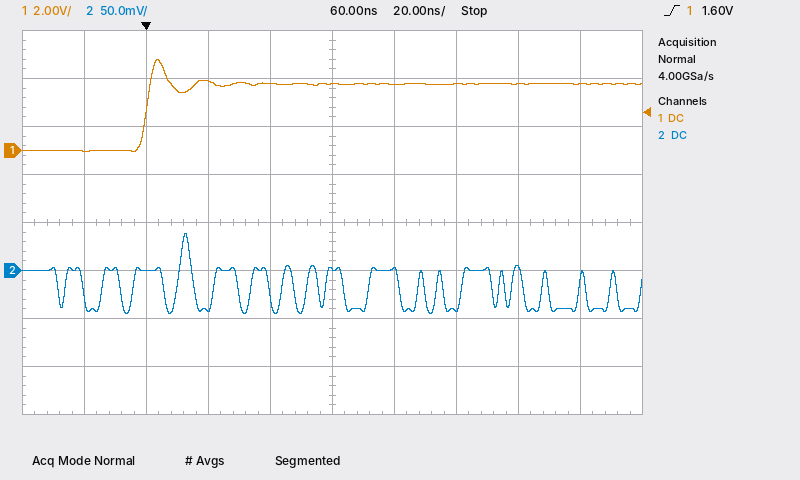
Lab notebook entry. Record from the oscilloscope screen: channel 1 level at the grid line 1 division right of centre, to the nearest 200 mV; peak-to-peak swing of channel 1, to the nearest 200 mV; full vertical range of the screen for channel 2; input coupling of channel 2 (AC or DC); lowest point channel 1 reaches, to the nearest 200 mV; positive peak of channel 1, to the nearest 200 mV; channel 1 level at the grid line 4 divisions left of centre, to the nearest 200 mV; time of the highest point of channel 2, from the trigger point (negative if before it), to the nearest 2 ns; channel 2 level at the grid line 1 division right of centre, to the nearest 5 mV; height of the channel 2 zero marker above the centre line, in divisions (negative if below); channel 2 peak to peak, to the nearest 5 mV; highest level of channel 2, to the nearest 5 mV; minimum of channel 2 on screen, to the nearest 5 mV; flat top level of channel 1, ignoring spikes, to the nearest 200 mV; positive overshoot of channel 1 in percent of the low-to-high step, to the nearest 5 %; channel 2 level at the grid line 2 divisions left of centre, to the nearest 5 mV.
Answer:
2.8 V
3.8 V
400 mV
DC
0.0 V
3.8 V
0.0 V
+12 ns
0 mV
-1.0 div
85 mV
40 mV
-45 mV
2.8 V
35 %
-40 mV
